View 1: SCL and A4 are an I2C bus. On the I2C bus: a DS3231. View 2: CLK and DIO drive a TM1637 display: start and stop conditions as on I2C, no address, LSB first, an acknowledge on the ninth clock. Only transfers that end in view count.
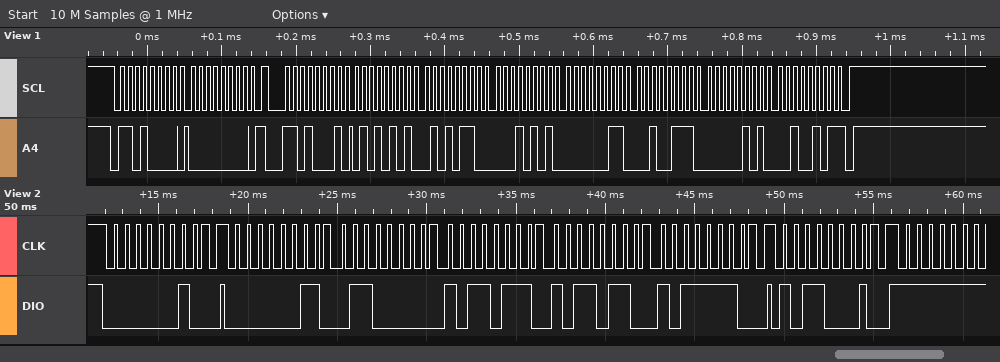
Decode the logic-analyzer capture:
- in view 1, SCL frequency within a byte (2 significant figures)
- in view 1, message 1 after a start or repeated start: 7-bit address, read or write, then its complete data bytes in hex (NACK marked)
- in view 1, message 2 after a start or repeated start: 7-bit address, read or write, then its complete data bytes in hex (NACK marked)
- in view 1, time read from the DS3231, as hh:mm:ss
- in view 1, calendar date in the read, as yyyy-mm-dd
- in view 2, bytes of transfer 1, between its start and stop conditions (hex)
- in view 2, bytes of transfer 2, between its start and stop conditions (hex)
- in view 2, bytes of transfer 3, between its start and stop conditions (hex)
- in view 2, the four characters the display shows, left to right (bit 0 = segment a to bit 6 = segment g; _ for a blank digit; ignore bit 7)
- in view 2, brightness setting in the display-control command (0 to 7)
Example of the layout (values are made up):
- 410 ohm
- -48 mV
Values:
- 100 kHz
- 0x68 write: 00
- 0x68 read: 55 56 15 03 27 05 25 NACK
- 15:56:55
- 2025-05-27
- 40
- C0 06 ED 6D 7D
- 8D
- 1556
- 5
